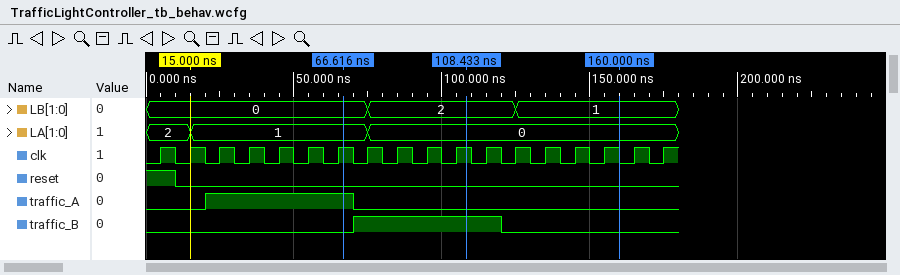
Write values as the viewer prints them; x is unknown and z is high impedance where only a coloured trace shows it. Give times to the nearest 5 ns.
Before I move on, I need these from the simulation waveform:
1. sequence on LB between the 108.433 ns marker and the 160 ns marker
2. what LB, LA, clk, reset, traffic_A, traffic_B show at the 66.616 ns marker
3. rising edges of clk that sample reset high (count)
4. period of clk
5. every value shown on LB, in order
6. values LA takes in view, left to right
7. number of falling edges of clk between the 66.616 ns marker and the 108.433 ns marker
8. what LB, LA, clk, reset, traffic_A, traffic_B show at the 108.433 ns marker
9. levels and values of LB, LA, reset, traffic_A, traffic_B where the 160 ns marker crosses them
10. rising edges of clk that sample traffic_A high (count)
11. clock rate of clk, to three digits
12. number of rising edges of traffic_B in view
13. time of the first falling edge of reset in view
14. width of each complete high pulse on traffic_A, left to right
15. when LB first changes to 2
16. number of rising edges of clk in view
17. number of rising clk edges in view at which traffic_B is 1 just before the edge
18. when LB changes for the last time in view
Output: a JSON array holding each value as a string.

["2, 1", "LB=0, LA=1, clk=1, reset=0, traffic_A=1, traffic_B=0", "1", "10 ns", "0, 2, 1", "2, 1, 0", "4", "LB=2, LA=0, clk=1, reset=0, traffic_A=0, traffic_B=1", "LB=1, LA=0, reset=0, traffic_A=0, traffic_B=0", "5", "100 MHz", "1", "10 ns", "50 ns", "75 ns", "18", "5", "125 ns"]
